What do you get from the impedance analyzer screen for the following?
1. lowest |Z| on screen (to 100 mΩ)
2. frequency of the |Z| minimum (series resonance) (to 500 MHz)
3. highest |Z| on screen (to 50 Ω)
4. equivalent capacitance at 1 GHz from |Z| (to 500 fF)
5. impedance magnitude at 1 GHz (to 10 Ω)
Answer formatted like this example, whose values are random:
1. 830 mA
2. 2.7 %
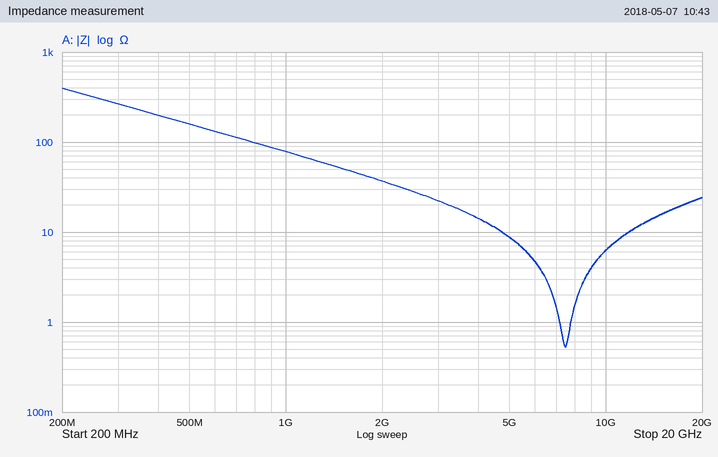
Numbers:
1. 500 mΩ
2. 7.5 GHz
3. 400 Ω
4. 2.0 pF
5. 80 Ω
